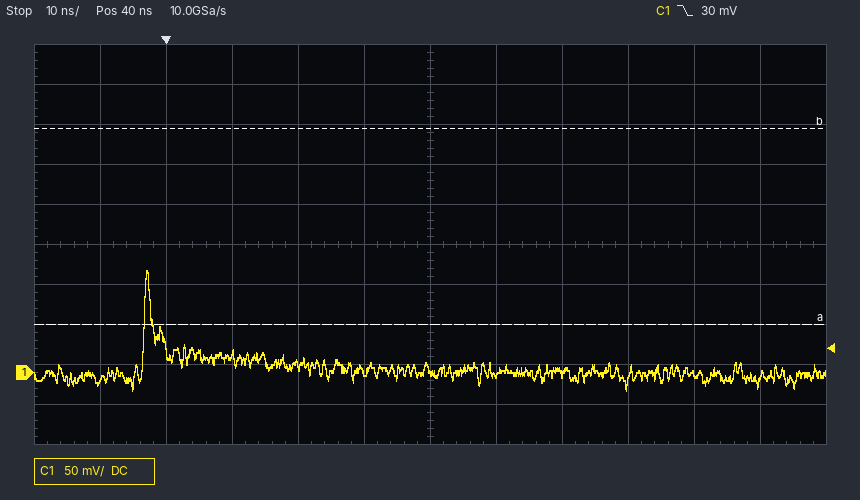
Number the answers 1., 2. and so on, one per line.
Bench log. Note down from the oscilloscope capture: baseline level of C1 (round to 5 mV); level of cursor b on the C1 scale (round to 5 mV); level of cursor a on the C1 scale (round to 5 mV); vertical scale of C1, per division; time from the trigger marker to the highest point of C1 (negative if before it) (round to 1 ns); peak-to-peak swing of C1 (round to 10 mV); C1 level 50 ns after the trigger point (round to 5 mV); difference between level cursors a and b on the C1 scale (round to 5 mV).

1. 0 mV
2. 305 mV
3. 60 mV
4. 50 mV
5. -3 ns
6. 150 mV
7. -5 mV
8. 245 mV
